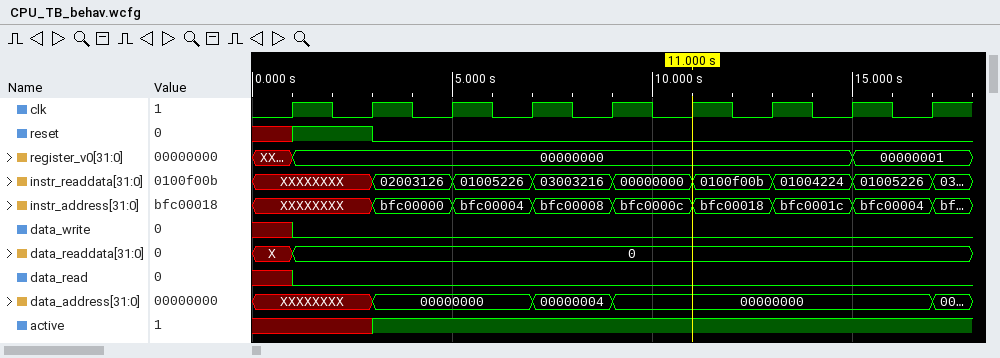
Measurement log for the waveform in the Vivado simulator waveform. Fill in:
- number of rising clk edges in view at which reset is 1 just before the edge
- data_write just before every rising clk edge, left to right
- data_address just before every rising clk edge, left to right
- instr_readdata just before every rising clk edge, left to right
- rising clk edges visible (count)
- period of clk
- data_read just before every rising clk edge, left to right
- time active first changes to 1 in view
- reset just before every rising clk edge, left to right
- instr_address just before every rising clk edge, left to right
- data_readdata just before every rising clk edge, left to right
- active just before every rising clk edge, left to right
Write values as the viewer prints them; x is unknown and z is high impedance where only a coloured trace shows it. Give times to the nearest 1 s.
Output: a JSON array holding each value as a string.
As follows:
["1", "x 0 0 0 0 0 0 0 0", "XXXXXXXX, XXXXXXXX, 00000000, 00000000, 00000004, 00000000, 00000000, 00000000, 00000000", "XXXXXXXX, XXXXXXXX, 02003126, 01005226, 03003216, 00000000, 0100f00b, 01004224, 01005226", "9", "2 s", "x 0 0 0 0 0 0 0 0", "3 s", "x 1 0 0 0 0 0 0 0", "XXXXXXXX, XXXXXXXX, bfc00000, bfc00004, bfc00008, bfc0000c, bfc00018, bfc0001c, bfc00004", "X, 0, 0, 0, 0, 0, 0, 0, 0", "x x 1 1 1 1 1 1 1"]
